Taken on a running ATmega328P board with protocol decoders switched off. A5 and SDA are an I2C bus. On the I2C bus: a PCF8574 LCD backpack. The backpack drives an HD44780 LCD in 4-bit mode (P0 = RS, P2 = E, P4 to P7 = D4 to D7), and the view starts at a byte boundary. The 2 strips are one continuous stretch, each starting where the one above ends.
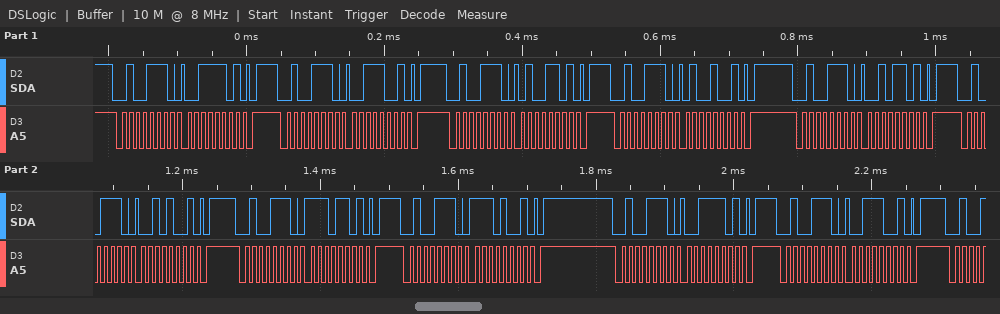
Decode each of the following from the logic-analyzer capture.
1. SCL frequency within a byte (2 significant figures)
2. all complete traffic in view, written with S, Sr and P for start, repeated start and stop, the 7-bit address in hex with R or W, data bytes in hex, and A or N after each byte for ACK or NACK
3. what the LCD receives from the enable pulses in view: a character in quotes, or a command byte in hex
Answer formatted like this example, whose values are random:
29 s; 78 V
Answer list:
100 kHz; S 27W A 3D A P S 27W A 39 A P S 27W A 4D A P S 27W A 49 A P S 27W A 2D A P S 27W A 29 A P S 27W A ED A P S 27W A E9 A P S 27W A 3D A P S 27W A 39 A P; '4' '.'
